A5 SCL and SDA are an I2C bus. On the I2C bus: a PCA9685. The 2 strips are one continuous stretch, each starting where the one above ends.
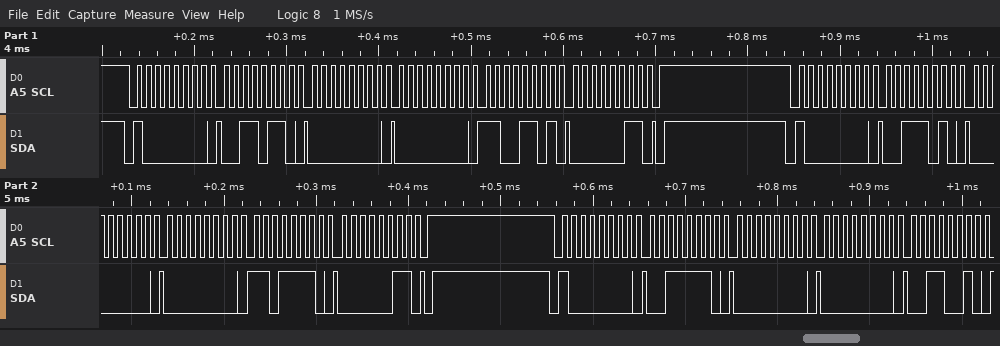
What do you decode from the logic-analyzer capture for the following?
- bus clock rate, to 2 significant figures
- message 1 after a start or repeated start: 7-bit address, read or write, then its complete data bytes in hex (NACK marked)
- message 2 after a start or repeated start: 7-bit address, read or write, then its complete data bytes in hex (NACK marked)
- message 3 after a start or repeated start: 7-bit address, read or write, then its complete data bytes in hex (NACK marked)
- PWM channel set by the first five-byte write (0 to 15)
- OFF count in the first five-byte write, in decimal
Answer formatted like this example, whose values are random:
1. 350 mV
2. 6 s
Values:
1. 100 kHz
2. 0x40 write: 36 00 00 CD 03
3. 0x40 write: 3A 00 00 DE 03
4. 0x40 write: 3E 00 00 32
5. 12
6. 973
